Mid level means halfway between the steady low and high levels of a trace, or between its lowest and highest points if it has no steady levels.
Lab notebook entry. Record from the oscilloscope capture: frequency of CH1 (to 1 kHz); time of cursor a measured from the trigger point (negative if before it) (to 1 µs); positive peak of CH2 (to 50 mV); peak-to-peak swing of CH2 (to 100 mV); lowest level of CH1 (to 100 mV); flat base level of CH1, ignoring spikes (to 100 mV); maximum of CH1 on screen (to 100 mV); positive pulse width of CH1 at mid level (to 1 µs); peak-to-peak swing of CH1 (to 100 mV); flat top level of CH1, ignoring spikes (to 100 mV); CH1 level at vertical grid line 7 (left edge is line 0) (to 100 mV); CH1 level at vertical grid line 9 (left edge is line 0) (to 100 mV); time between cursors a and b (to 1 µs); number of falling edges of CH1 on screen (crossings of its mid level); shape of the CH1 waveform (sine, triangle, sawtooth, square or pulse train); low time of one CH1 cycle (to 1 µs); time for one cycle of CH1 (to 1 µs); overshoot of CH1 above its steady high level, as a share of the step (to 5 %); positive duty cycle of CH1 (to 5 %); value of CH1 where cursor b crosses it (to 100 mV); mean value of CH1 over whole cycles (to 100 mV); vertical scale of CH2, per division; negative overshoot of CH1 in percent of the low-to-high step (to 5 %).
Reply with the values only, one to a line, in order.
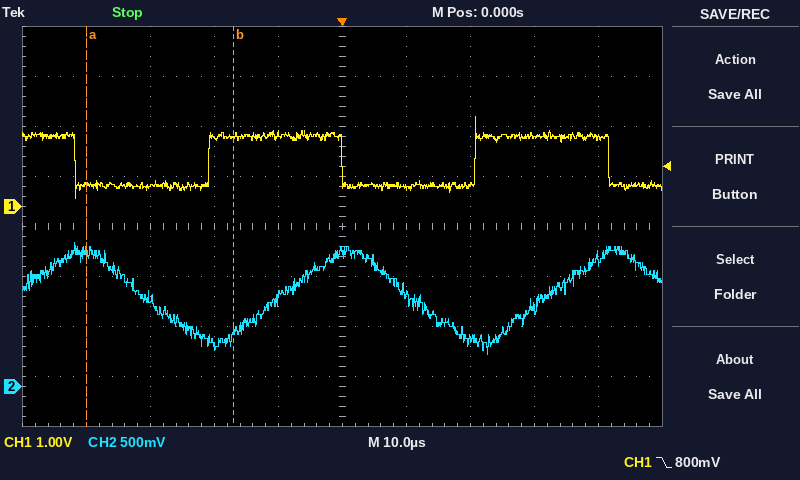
24 kHz
-40 µs
1.45 V
1.10 V
200 mV
400 mV
1.8 V
21 µs
1.6 V
1.4 V
400 mV
1.4 V
23 µs
3
square
21 µs
42 µs
40 %
50 %
1.4 V
900 mV
500 mV
25 %
